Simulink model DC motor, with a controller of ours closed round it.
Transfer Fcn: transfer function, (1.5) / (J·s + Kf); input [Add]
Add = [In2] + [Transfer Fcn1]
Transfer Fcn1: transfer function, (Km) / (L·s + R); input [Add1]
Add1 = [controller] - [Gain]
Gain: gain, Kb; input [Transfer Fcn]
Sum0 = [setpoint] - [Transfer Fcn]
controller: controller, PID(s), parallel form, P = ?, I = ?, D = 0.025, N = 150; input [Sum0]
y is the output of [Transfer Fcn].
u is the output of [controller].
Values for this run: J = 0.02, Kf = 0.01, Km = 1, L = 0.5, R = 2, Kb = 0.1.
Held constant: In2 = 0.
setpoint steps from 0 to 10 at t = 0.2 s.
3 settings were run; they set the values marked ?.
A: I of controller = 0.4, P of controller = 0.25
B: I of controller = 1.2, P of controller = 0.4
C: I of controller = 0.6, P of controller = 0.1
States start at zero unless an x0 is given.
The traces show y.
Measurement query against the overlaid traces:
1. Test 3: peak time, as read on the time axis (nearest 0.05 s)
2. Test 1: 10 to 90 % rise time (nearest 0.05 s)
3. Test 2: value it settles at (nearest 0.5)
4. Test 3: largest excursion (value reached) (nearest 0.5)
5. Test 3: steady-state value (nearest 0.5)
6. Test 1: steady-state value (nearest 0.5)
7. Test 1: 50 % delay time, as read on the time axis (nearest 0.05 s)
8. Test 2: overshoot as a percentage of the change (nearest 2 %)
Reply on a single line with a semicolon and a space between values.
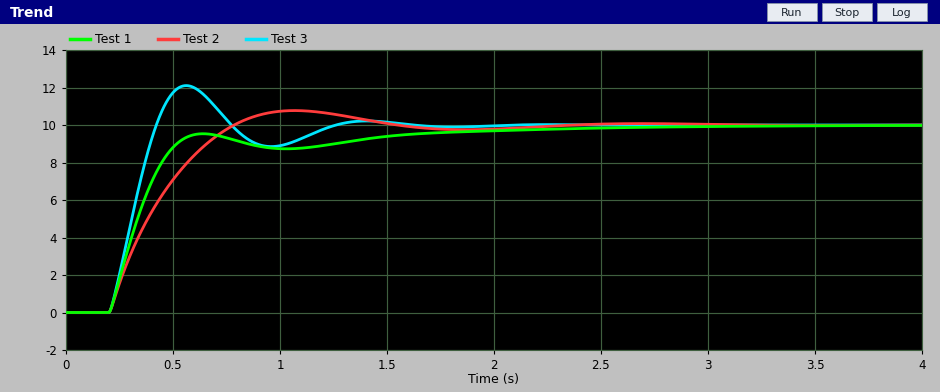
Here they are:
0.55 s; 0.30 s; 10.0; 12.0; 10.0; 10.0; 0.35 s; 8 %
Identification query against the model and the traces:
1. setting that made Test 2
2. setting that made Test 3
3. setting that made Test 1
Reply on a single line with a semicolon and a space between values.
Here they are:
C; B; A
